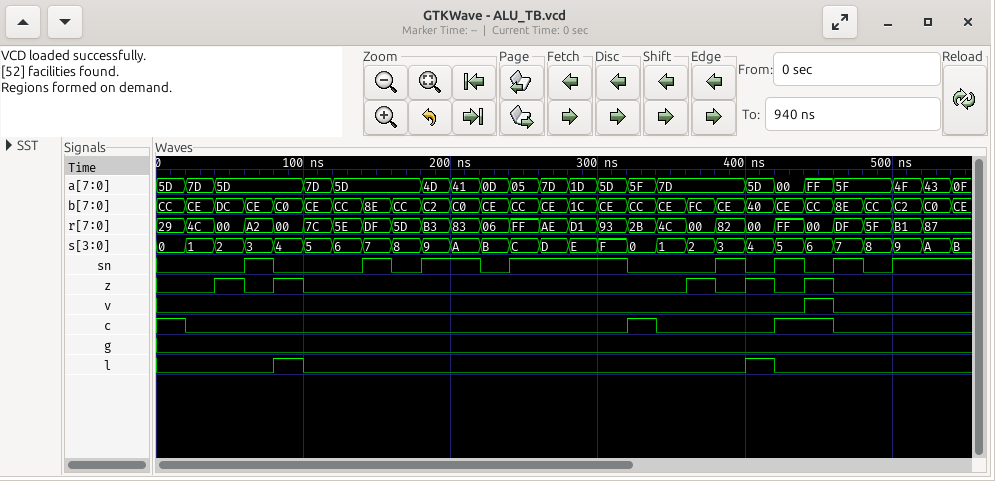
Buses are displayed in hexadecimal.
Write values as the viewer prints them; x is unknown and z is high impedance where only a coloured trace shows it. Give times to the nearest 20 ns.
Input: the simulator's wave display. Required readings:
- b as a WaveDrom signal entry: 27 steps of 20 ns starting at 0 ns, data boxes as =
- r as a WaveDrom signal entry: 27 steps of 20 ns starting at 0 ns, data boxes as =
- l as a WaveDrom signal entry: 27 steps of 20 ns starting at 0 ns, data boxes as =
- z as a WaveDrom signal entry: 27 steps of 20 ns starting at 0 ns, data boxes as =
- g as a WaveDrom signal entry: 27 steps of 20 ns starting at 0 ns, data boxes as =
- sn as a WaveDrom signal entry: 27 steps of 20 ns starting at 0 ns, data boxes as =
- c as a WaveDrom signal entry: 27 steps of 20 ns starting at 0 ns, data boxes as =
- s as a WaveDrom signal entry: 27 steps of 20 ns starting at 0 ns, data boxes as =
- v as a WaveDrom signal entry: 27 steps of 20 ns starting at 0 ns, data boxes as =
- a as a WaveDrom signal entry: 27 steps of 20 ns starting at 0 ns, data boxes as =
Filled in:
{name: 'b', wave: '===========================', data: 'CC CE DC CE C0 CE CC 8E CC C2 C0 CE CC CE 1C CE CC CE FC CE 40 CE CC 8E CC C2 C0'}
{name: 'r', wave: '===========================', data: '29 4C 00 A2 00 7C 5E DF 5D B3 83 06 FF AE D1 93 2B 4C 00 82 00 FF 00 DF 5F B1 87'}
{name: 'l', wave: '0...10..............10.....'}
{name: 'z', wave: '0.1010............101010...'}
{name: 'g', wave: '0..........................'}
{name: 'sn', wave: '0..10..101.01...0..1010101.'}
{name: 'c', wave: '10..............10...1.0...'}
{name: 's', wave: '===========================', data: '0 1 2 3 4 5 6 7 8 9 A B C D E F 0 1 2 3 4 5 6 7 8 9 A'}
{name: 'v', wave: '0.....................10...'}
{name: 'a', wave: '===..==..=========..====.==', data: '5D 7D 5D 7D 5D 4D 41 0D 05 7D 1D 5D 5F 7D 5D 00 FF 5F 4F 43'}
